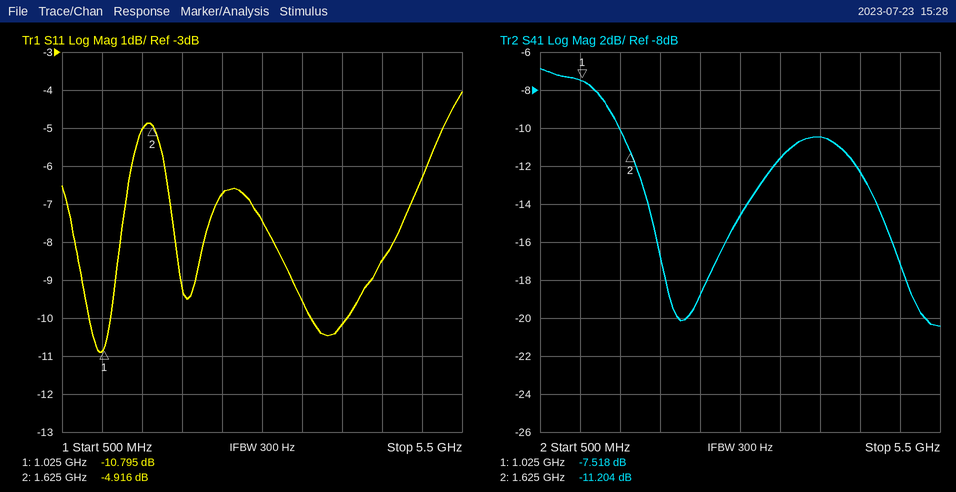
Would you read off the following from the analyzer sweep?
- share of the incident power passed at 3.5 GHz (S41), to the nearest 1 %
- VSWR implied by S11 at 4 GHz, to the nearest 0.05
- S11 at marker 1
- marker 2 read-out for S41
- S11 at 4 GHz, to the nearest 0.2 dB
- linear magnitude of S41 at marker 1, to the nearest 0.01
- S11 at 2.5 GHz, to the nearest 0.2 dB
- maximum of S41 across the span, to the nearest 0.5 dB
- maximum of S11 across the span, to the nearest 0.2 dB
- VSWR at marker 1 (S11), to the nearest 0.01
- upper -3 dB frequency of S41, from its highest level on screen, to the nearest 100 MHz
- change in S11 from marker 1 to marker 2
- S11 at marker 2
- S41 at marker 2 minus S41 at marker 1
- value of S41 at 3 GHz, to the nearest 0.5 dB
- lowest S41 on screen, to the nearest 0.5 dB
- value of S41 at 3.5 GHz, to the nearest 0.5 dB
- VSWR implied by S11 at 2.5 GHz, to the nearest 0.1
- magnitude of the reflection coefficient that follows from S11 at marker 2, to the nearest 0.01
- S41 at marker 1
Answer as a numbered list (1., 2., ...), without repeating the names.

1. 7 %
2. 1.90
3. -10.795 dB
4. -11.204 dB
5. -10.2 dB
6. 0.42
7. -6.8 dB
8. -7.0 dB
9. -4.0 dB
10. 1.81
11. 1.5 GHz
12. 5.879 dB
13. -4.916 dB
14. -3.686 dB
15. -14.5 dB
16. -20.5 dB
17. -11.5 dB
18. 2.7
19. 0.57
20. -7.518 dB
